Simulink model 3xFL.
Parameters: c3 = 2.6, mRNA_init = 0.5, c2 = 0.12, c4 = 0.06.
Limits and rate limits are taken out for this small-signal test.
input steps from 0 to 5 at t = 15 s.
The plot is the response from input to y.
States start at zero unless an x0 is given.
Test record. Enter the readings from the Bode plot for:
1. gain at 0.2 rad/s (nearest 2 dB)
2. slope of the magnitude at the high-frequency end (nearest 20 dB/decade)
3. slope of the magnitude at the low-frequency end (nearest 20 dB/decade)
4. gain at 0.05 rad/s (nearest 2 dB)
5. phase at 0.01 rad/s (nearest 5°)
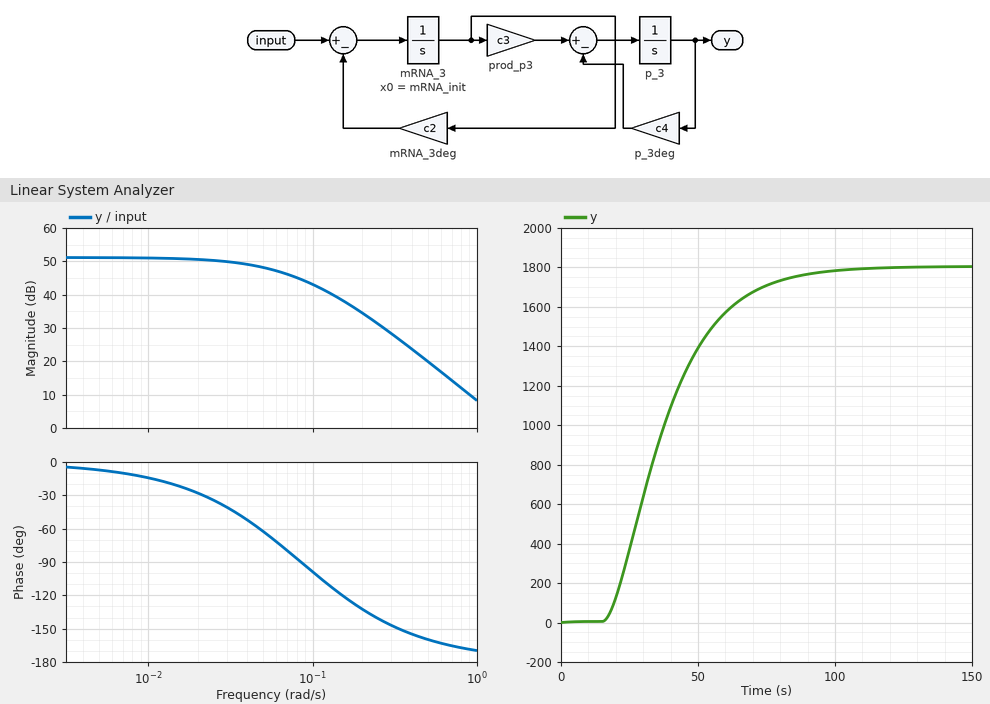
34 dB
-40 dB/decade
0 dB/decade
48 dB
-15°
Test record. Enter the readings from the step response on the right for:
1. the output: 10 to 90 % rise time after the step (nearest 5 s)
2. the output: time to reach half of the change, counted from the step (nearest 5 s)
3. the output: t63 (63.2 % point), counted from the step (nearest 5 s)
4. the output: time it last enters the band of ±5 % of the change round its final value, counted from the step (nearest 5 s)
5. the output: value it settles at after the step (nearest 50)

45 s
20 s
25 s
60 s
1800
